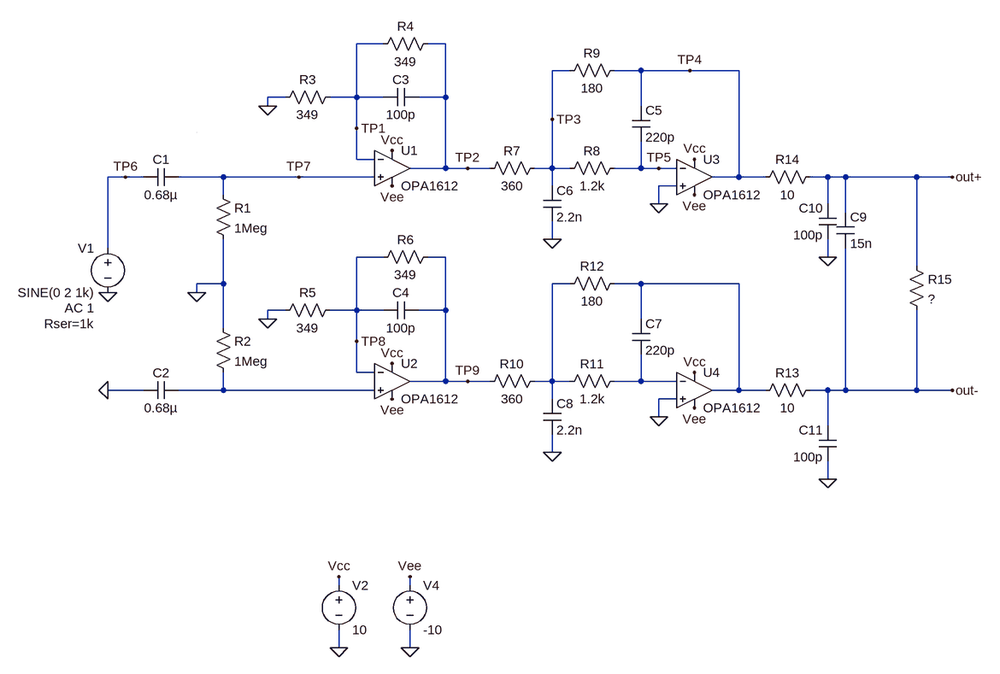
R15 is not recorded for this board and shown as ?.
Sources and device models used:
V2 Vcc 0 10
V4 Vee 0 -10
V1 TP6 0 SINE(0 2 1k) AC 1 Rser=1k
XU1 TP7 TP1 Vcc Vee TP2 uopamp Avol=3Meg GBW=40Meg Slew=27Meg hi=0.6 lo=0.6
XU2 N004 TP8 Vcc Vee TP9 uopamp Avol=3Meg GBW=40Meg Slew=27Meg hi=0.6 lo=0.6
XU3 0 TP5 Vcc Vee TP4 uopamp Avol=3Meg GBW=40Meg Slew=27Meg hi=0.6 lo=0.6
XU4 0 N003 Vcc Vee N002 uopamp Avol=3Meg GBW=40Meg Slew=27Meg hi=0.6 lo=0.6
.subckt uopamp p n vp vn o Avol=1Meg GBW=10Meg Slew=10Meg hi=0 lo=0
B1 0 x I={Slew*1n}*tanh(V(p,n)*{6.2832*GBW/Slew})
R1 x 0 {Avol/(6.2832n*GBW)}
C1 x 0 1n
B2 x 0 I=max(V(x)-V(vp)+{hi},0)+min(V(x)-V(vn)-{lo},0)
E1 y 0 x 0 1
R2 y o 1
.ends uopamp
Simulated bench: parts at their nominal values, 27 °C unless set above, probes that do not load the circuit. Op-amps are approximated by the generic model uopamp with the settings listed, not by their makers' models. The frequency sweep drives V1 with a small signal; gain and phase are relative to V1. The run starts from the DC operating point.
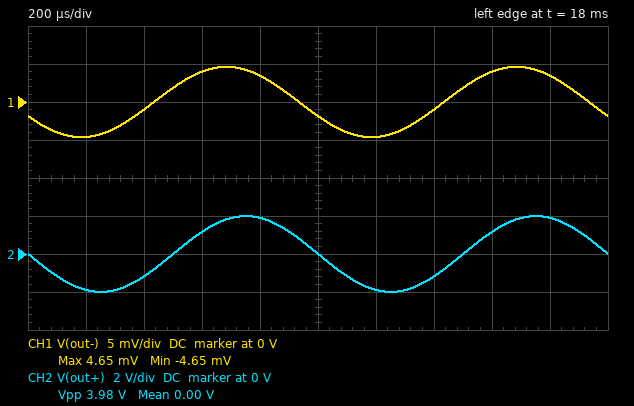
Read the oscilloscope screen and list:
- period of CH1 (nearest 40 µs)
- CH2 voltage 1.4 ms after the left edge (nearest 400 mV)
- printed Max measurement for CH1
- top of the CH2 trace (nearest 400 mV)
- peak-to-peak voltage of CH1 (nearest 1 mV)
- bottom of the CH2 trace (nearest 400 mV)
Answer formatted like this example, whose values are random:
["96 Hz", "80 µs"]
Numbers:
["1.00 ms", "-1.2 V", "4.65 mV", "2.0 V", "9 mV", "-2.0 V"]
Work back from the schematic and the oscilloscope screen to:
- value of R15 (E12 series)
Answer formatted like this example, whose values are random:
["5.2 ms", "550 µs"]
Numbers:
["4.7 kΩ"]
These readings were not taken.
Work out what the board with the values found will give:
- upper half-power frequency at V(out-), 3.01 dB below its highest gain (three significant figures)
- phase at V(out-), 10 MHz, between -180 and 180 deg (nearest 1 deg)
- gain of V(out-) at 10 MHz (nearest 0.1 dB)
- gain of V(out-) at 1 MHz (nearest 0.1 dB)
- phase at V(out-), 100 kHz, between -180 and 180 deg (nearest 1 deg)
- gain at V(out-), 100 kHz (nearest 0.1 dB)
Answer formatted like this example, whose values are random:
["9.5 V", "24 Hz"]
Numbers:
["685 kHz", "-44 deg", "-63.8 dB", "-19.8 dB", "-119 deg", "-20.7 dB"]
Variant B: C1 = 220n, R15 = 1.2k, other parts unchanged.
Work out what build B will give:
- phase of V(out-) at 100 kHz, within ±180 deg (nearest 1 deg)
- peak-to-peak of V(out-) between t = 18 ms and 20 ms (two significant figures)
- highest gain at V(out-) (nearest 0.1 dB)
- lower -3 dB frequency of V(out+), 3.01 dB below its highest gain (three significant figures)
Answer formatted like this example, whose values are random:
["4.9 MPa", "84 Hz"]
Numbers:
["-123 deg", "33 mV", "-11.8 dB", "723 mHz"]
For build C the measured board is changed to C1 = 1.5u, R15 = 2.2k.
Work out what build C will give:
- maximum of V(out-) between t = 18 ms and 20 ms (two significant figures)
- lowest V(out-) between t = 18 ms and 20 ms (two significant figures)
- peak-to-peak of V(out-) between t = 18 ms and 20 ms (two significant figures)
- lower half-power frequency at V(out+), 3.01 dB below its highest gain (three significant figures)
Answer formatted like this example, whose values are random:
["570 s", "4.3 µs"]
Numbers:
["9.2 mV", "-9.2 mV", "18 mV", "106 mHz"]
